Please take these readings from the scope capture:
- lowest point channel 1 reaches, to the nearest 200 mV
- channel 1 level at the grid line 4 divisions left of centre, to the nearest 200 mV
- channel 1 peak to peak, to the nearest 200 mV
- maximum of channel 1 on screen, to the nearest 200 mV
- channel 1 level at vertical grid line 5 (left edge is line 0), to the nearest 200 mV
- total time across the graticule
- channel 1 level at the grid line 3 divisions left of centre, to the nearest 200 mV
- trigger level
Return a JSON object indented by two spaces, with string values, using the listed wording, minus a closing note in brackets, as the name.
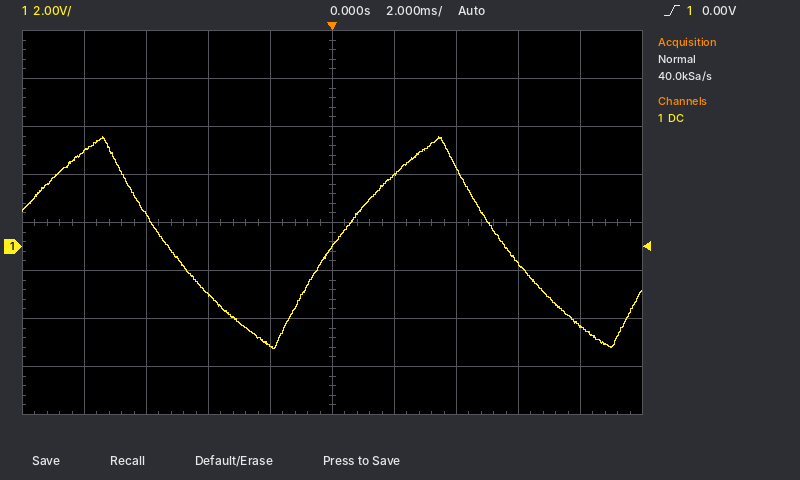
{
  "lowest point channel 1 reaches, to the nearest 200 mV": "-4.2 V",
  "channel 1 level at the grid line 4 divisions left of centre, to the nearest 200 mV": "4.0 V",
  "channel 1 peak to peak, to the nearest 200 mV": "8.8 V",
  "maximum of channel 1 on screen, to the nearest 200 mV": "4.6 V",
  "channel 1 level at vertical grid line 5 (left edge is line 0), to the nearest 200 mV": "0.0 V",
  "total time across the graticule": "20 ms",
  "channel 1 level at the grid line 3 divisions left of centre, to the nearest 200 mV": "1.4 V",
  "trigger level": "0.00 V"
}
